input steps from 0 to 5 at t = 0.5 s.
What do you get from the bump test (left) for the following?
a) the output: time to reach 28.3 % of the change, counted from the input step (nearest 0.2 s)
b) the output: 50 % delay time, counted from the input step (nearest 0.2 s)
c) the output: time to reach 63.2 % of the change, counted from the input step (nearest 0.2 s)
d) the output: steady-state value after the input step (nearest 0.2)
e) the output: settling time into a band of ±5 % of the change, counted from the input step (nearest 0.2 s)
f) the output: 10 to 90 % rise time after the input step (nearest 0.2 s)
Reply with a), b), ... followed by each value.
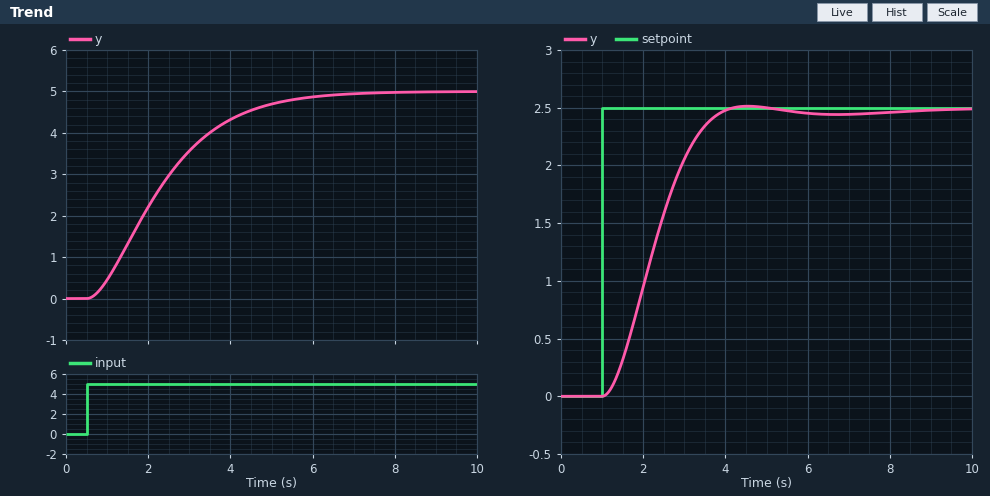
a) 1.0 s
b) 1.6 s
c) 2.2 s
d) 5.0
e) 4.8 s
f) 3.4 s
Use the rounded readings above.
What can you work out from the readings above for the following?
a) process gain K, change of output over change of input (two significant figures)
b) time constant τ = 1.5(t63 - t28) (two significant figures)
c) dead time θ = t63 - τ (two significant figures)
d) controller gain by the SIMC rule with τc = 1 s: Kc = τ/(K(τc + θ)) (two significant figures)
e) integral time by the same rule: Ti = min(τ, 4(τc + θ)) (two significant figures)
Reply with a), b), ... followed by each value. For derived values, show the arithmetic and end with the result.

a) (5 - 0) / 5 = 1.0
b) 1.5 × (2.2 - 1) = 1.8 s
c) 2.2 - 1.8 = 0.40 s
d) 1.8 / (1 × (1 + 0.4)) = 1.3
e) min(1.8, 4 × (1 + 0.4)) = 1.8 s
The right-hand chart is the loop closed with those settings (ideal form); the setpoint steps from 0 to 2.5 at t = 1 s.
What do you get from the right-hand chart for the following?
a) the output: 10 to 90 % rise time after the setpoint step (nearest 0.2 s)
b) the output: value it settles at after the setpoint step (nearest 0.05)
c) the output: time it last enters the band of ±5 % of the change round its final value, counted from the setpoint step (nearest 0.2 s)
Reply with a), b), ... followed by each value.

a) 1.8 s
b) 2.50
c) 2.6 s
